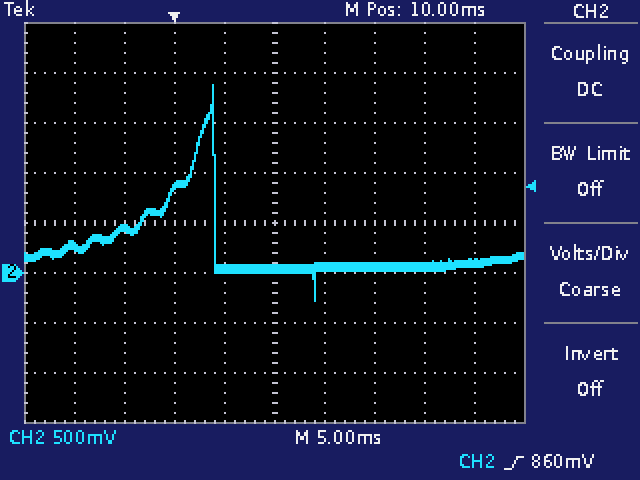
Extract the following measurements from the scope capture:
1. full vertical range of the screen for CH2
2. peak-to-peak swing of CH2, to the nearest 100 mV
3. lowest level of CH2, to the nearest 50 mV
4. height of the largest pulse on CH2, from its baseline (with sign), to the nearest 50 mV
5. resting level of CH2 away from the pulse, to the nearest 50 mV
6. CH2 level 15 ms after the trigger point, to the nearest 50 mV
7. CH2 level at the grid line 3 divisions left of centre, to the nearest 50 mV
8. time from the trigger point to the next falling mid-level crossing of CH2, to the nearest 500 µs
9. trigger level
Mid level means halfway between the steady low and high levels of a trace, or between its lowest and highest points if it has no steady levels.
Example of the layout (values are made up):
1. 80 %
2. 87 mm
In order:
1. 4 V
2. 2.20 V
3. -300 mV
4. +1.80 V
5. 50 mV
6. 50 mV
7. 450 mV
8. 4.0 ms
9. 860 mV
